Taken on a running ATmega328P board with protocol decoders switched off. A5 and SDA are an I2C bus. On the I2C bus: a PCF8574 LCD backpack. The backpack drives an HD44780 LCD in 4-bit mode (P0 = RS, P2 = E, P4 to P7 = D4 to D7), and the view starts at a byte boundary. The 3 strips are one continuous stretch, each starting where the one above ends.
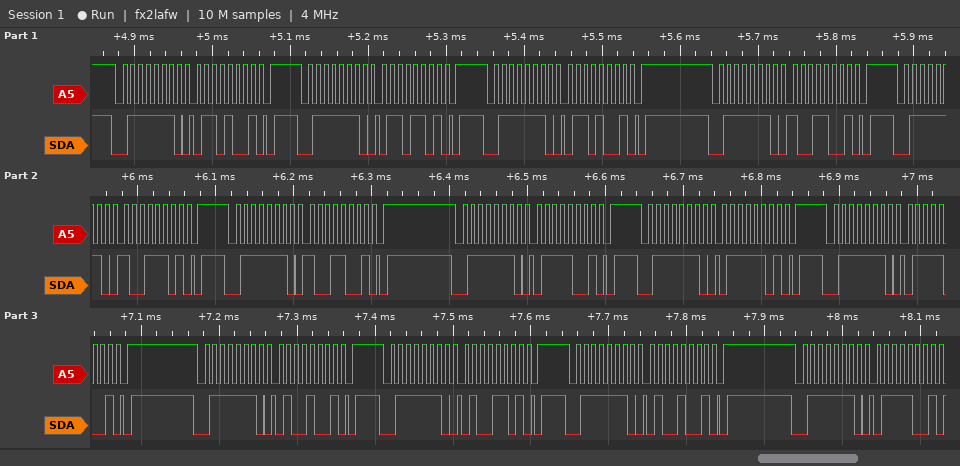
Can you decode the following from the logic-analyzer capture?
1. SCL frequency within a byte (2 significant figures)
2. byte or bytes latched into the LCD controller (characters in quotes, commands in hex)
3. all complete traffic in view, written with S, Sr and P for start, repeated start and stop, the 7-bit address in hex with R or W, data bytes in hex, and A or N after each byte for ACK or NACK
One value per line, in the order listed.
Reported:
100 kHz
'i' 't'
S 3FW A 69 A P S 3FW A 6D A P S 3FW A 69 A P S 3FW A 99 A P S 3FW A 9D A P S 3FW A 99 A P S 3FW A 79 A P S 3FW A 7D A P S 3FW A 79 A P S 3FW A 49 A P S 3FW A 4D A P S 3FW A 49 A P S 3FW A 79 A
